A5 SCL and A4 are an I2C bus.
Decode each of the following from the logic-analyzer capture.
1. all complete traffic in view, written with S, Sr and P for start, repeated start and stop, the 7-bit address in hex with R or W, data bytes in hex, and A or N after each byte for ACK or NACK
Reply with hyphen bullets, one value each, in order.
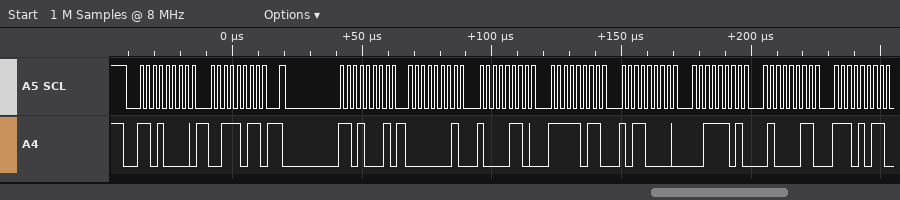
- S 68W A 3B A Sr 68R A 01 A 86 A FB A B0 A 3D A 43 A EB A
